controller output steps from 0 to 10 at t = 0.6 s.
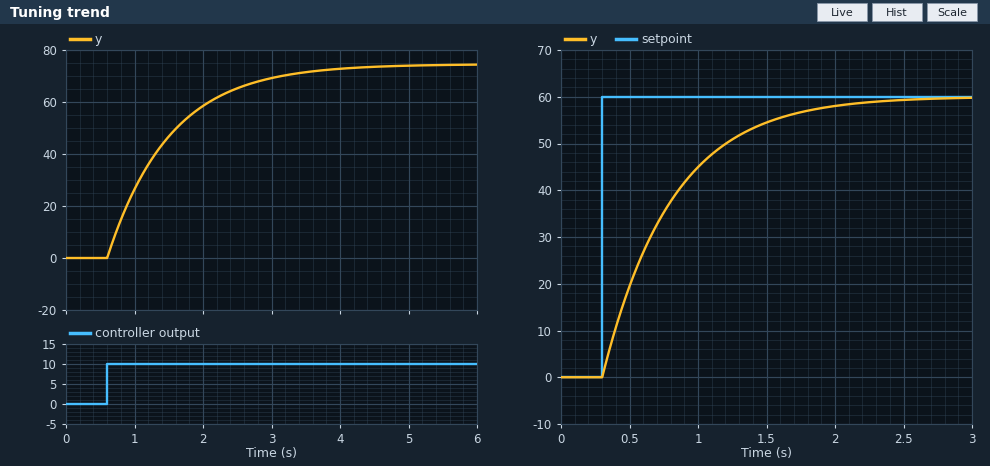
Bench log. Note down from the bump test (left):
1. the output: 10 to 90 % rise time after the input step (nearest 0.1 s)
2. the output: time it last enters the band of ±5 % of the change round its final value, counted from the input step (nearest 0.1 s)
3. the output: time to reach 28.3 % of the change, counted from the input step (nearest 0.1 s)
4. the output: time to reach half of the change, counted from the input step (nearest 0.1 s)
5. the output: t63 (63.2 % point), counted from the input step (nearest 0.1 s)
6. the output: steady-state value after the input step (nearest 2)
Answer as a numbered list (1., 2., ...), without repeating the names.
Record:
1. 2.0 s
2. 2.7 s
3. 0.3 s
4. 0.6 s
5. 0.9 s
6. 74
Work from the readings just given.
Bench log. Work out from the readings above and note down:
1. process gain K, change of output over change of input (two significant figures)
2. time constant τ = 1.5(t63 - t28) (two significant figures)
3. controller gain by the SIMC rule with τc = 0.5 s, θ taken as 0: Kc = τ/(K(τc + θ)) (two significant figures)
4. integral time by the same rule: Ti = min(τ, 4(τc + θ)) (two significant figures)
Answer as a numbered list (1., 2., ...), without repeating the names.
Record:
1. 7.4
2. 0.90 s
3. 0.24
4. 0.90 s
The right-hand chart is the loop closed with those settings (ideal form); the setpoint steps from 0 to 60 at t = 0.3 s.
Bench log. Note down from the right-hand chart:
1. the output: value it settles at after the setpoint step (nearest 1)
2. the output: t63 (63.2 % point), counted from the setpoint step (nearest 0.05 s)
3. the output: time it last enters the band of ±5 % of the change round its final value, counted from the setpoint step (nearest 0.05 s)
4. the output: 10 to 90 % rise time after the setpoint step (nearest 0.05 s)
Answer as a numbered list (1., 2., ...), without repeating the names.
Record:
1. 60
2. 0.50 s
3. 1.50 s
4. 1.10 s
